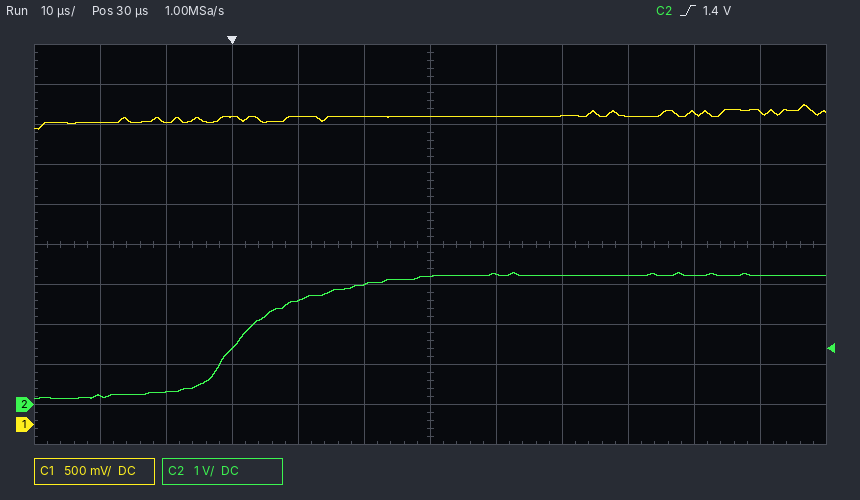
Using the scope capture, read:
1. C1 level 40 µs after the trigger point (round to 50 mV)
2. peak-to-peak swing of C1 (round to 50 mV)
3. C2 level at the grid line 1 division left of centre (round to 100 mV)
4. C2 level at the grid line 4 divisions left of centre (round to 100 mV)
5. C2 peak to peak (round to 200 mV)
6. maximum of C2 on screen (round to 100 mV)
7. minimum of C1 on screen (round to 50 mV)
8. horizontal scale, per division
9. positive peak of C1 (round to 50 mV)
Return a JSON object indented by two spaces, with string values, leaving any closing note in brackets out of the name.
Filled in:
{
  "C1 level 40 µs after the trigger point": "3.85 V",
  "peak-to-peak swing of C1": "300 mV",
  "C2 level at the grid line 1 division left of centre": "3.0 V",
  "C2 level at the grid line 4 divisions left of centre": "300 mV",
  "C2 peak to peak": "3.2 V",
  "maximum of C2 on screen": "3.3 V",
  "minimum of C1 on screen": "3.70 V",
  "horizontal scale, per division": "10 µs",
  "positive peak of C1": "4.00 V"
}
